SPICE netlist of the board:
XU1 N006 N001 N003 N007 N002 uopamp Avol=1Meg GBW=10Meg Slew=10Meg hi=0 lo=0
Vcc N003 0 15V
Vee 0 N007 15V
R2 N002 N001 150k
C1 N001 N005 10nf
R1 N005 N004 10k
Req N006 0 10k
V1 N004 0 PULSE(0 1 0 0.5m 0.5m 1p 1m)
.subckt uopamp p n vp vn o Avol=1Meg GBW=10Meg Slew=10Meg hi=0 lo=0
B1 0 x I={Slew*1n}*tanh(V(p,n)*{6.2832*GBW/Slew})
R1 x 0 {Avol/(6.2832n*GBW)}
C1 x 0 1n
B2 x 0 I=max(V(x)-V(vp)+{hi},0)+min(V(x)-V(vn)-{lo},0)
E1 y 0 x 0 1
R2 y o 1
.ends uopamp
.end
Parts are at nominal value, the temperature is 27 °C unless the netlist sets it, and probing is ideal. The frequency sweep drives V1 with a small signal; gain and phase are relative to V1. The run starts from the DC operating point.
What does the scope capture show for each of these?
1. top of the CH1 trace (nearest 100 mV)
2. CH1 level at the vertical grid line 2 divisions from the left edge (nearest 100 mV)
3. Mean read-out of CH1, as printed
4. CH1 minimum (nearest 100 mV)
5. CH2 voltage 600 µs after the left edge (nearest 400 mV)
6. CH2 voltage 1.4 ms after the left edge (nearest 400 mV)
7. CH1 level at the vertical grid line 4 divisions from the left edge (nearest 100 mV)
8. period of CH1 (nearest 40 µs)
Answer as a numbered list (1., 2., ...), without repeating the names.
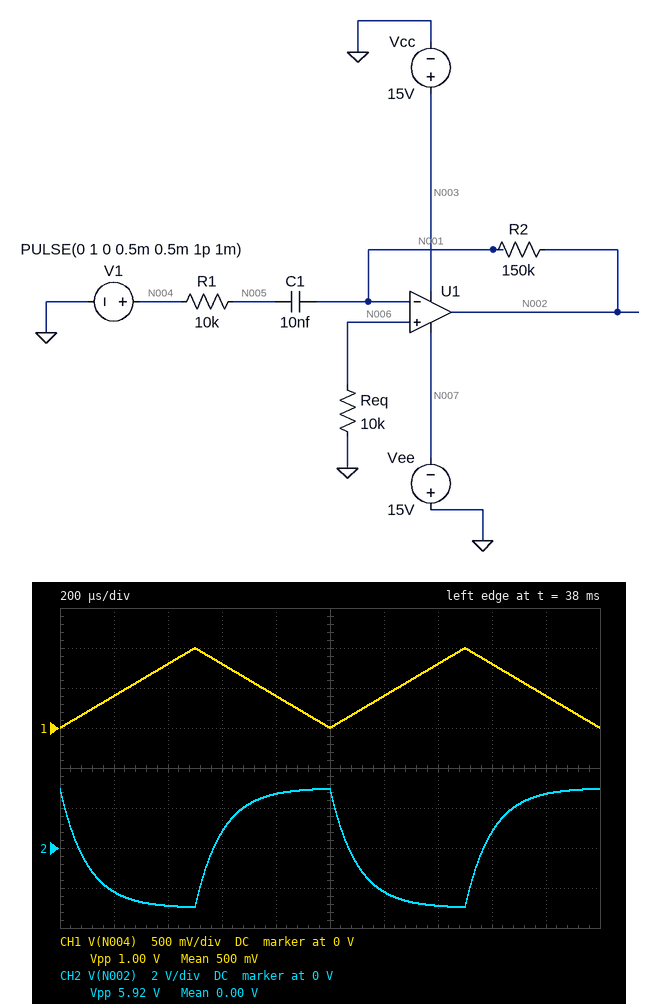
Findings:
1. 1.0 V
2. 800 mV
3. 500 mV
4. 0 V
5. 800 mV
6. -2.8 V
7. 400 mV
8. 1.00 ms
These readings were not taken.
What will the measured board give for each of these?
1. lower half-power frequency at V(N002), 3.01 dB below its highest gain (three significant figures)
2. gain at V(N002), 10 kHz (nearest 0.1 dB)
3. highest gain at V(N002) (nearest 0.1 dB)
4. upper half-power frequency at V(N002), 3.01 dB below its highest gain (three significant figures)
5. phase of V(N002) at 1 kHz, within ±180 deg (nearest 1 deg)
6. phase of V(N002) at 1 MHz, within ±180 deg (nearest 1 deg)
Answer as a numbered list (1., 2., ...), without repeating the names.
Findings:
1. 1.59 kHz
2. 23.4 dB
3. 23.5 dB
4. 627 kHz
5. -122 deg
6. 122 deg
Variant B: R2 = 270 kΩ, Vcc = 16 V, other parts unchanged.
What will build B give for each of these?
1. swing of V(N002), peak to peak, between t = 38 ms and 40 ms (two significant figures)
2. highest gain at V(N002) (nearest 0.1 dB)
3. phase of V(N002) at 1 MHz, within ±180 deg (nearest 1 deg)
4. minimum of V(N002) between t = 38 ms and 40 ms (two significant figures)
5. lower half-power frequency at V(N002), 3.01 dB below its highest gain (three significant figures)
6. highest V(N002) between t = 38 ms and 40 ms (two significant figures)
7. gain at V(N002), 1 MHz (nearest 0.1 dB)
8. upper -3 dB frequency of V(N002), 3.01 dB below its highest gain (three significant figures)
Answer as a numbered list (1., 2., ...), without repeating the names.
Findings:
1. 11 V
2. 28.6 dB
3. 110 deg
4. -5.3 V
5. 1.58 kHz
6. 5.3 V
7. 19.2 dB
8. 359 kHz
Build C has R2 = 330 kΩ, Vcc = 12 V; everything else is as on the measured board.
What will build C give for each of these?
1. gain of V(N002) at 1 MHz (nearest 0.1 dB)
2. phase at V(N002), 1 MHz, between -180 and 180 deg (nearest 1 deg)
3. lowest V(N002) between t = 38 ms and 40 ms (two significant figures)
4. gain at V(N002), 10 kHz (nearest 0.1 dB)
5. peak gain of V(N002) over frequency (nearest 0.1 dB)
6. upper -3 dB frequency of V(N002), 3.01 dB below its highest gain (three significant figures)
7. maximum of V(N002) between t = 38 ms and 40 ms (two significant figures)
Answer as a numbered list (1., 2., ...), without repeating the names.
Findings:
1. 19.4 dB
2. 106 deg
3. -6.5 V
4. 30.3 dB
5. 30.4 dB
6. 296 kHz
7. 6.5 V
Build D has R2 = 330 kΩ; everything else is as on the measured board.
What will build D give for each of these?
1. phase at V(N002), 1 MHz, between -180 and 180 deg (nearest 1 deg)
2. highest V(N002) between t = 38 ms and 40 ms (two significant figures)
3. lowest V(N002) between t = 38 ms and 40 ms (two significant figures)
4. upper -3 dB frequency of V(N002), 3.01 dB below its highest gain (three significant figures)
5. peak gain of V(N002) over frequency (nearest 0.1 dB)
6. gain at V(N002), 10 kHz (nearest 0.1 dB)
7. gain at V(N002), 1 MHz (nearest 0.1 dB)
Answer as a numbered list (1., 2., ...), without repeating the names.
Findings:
1. 106 deg
2. 6.5 V
3. -6.5 V
4. 296 kHz
5. 30.4 dB
6. 30.3 dB
7. 19.4 dB
